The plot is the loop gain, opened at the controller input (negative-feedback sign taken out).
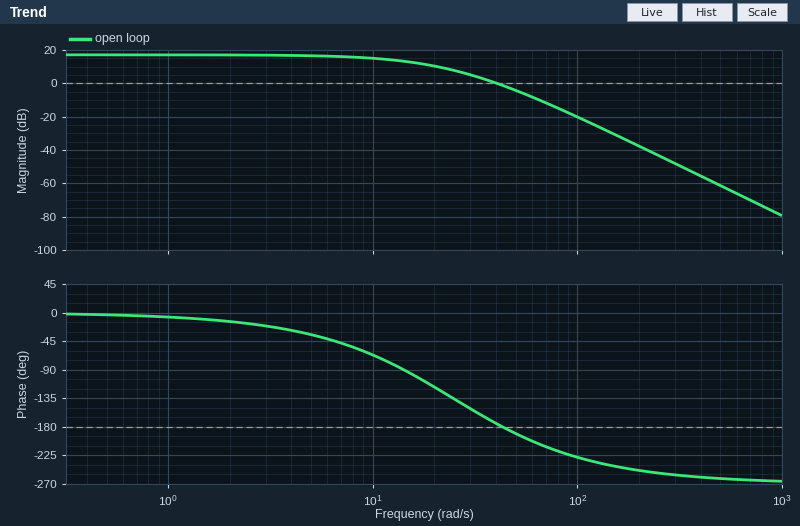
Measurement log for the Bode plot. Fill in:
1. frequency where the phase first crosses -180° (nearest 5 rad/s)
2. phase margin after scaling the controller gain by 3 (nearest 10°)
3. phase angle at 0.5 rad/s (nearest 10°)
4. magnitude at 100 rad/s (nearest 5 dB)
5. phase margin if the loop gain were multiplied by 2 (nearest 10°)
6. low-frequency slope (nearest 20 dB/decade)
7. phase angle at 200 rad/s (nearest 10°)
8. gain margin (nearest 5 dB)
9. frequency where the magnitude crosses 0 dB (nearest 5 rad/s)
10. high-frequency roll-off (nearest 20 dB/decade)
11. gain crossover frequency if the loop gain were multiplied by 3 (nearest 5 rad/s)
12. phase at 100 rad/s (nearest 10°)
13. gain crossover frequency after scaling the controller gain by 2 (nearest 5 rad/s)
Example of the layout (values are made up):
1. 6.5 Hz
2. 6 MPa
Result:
1. 45 rad/s
2. -30°
3. 0°
4. -20 dB
5. -20°
6. 0 dB/decade
7. -250°
8. 0 dB
9. 40 rad/s
10. -60 dB/decade
11. 65 rad/s
12. -230°
13. 55 rad/s
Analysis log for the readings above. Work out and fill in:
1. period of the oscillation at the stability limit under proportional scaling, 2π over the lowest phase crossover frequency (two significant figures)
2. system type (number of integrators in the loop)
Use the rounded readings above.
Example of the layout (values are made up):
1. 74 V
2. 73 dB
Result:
1. 0.14 s
2. 0
